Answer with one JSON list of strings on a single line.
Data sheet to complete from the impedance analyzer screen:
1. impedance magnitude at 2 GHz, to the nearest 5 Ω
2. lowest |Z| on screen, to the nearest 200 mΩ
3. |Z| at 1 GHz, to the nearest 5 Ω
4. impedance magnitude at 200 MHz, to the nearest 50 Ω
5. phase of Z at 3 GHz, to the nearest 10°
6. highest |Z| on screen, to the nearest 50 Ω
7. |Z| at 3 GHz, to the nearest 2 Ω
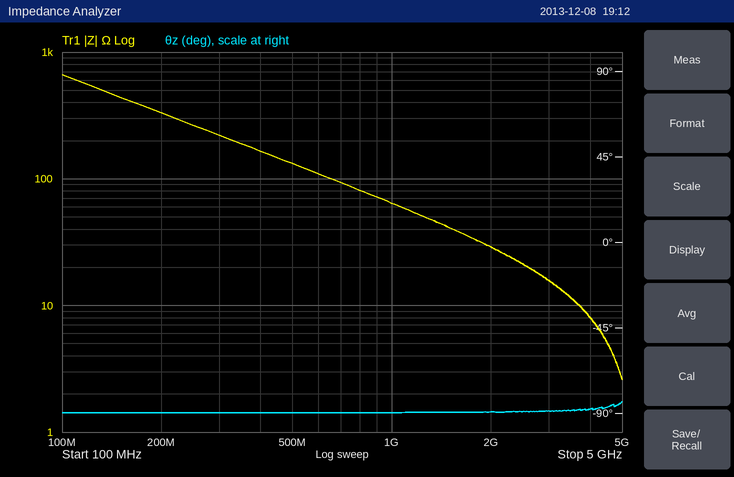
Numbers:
["30 Ω", "2.6 Ω", "65 Ω", "350 Ω", "-90°", "650 Ω", "16 Ω"]
